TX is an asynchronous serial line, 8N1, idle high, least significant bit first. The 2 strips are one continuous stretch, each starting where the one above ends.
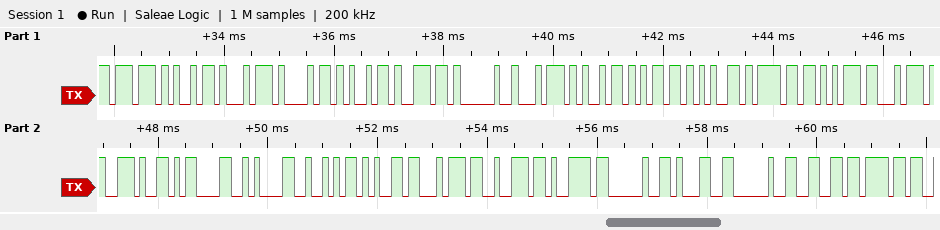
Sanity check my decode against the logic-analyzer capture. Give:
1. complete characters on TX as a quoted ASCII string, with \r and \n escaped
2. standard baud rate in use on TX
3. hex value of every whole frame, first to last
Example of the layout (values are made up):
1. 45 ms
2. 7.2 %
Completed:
1. "within timeout.\r\nRetry 1 fo"
2. 9600 baud
3. 77 69 74 68 69 6E 20 74 69 6D 65 6F 75 74 2E 0D 0A 52 65 74 72 79 20 31 20 66 6F
